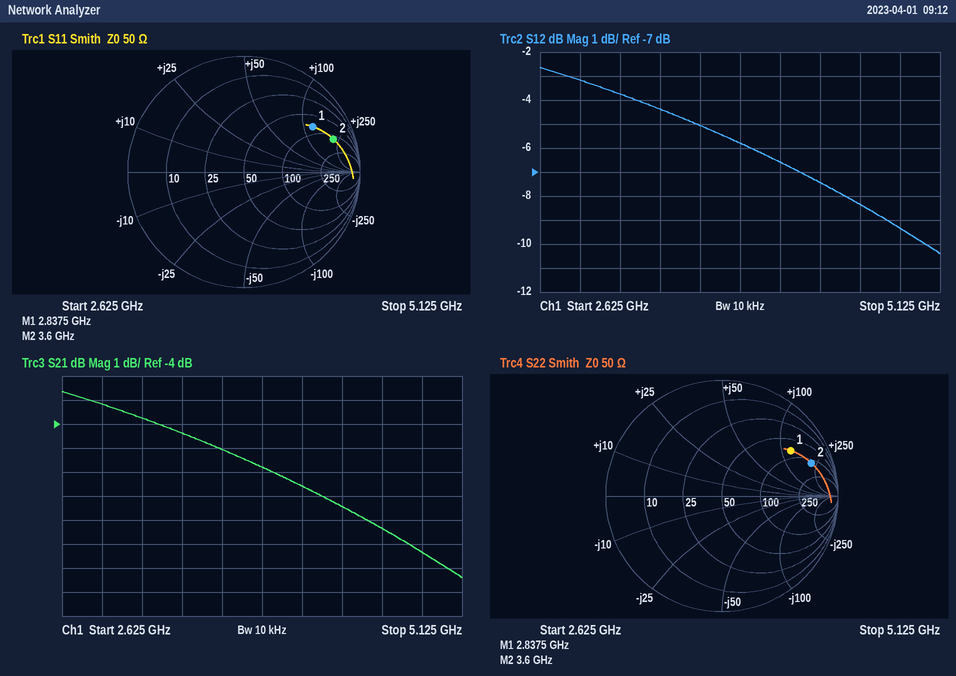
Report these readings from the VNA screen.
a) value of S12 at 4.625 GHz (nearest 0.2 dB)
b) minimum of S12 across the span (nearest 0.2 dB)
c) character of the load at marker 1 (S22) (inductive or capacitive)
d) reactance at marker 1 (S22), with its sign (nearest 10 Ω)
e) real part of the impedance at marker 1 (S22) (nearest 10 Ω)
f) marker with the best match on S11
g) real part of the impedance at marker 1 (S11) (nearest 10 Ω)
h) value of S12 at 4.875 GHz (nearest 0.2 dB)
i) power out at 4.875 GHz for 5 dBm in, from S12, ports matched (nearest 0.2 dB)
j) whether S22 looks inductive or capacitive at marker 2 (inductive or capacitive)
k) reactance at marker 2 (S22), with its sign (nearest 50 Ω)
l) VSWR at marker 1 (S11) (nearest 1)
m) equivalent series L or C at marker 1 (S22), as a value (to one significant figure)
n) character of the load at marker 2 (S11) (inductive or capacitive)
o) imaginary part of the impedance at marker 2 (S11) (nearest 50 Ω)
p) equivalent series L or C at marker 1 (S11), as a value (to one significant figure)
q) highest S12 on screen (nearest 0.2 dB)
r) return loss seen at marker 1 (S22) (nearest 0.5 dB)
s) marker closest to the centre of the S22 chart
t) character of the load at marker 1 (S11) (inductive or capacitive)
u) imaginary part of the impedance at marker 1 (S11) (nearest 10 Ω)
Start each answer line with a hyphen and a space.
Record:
- -8.4 dB
- -10.4 dB
- inductive
- +120 Ω
- 80 Ω
- marker 1
- 80 Ω
- -9.4 dB
- -4.4 dBm
- inductive
- +200 Ω
- 6
- 7 nH
- inductive
- +200 Ω
- 7 nH
- -2.6 dB
- 3.0 dB
- marker 1
- inductive
- +120 Ω
